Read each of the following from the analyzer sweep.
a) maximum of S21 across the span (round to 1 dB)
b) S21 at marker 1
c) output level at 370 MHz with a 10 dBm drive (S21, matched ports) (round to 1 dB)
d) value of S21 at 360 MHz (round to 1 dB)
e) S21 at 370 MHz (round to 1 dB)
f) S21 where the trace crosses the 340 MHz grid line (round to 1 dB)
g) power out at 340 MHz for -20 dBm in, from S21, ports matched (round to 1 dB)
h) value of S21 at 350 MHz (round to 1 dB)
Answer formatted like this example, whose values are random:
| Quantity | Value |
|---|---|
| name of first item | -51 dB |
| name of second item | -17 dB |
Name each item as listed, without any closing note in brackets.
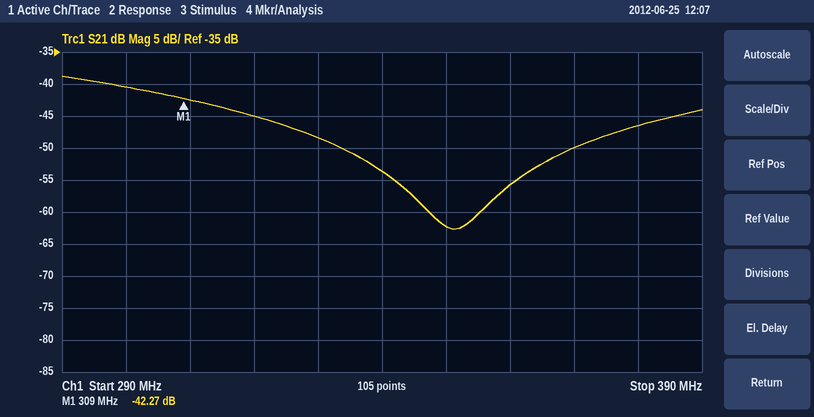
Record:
| Quantity | Value |
|---|---|
| maximum of S21 across the span | -39 dB |
| S21 at marker 1 | -42.27 dB |
| output level at 370 MHz with a 10 dBm drive (S21, matched ports) | -40 dBm |
| value of S21 at 360 MHz | -56 dB |
| S21 at 370 MHz | -50 dB |
| S21 where the trace crosses the 340 MHz grid line | -54 dB |
| power out at 340 MHz for -20 dBm in, from S21, ports matched | -74 dBm |
| value of S21 at 350 MHz | -62 dB |
